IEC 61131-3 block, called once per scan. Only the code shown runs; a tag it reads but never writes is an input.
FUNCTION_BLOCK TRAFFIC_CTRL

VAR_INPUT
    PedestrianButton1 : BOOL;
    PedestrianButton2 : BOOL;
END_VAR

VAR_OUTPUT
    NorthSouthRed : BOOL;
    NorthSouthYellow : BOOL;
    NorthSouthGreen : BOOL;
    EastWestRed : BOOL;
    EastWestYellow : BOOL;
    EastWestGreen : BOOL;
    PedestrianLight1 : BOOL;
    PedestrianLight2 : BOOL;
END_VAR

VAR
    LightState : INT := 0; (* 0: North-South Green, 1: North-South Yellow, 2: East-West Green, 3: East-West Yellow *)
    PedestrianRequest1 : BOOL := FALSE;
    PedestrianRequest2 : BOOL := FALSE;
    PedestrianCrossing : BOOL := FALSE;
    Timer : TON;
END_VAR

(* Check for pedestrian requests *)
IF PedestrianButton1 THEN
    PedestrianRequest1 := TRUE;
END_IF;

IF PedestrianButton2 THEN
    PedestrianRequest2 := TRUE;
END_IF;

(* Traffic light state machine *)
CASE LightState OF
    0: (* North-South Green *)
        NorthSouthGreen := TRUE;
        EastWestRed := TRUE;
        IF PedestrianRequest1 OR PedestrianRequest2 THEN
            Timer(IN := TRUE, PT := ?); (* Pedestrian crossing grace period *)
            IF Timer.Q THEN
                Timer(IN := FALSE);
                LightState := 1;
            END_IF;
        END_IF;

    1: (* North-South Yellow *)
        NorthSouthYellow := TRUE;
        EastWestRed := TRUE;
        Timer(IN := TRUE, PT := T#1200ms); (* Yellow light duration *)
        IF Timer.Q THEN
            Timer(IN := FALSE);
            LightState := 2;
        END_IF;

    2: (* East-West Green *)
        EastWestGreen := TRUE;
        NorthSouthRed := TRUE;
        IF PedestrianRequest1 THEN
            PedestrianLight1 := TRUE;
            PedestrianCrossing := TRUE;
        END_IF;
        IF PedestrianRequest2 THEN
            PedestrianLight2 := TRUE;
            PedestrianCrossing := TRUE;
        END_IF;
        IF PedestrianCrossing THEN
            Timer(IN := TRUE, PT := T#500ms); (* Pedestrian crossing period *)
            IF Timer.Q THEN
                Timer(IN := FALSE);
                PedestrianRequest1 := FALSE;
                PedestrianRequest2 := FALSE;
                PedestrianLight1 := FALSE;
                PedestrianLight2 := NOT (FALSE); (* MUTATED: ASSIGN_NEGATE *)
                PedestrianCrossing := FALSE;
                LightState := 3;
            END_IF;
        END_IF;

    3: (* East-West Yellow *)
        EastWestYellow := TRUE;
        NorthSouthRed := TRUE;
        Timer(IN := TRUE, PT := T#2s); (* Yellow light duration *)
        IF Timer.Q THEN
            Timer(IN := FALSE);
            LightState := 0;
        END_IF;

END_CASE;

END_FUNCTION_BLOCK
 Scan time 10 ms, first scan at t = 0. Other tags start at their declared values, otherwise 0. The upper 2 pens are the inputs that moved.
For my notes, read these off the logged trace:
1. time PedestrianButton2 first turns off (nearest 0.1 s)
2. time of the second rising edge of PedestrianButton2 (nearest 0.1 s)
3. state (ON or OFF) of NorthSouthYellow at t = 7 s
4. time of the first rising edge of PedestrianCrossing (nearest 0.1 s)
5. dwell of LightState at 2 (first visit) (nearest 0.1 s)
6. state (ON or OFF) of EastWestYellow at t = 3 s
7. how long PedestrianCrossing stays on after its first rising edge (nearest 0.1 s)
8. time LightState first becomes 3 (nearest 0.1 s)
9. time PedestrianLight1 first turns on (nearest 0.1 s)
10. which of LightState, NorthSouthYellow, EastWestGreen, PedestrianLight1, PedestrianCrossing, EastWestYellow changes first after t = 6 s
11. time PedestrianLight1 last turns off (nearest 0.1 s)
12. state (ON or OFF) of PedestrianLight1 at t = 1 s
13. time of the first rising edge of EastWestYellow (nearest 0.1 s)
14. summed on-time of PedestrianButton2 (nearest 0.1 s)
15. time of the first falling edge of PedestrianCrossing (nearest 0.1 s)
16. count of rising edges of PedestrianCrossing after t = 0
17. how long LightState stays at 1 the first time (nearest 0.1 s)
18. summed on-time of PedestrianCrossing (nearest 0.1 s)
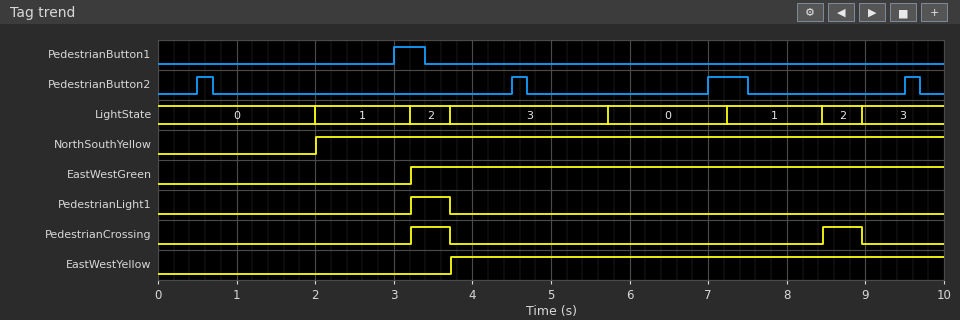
0.7 s
4.5 s
ON
3.2 s
0.5 s
OFF
0.5 s
3.7 s
3.2 s
LightState
3.7 s
OFF
3.7 s
1.1 s
3.7 s
2
1.2 s
1.0 s
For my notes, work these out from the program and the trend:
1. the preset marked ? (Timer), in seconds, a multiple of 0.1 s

1.5 s
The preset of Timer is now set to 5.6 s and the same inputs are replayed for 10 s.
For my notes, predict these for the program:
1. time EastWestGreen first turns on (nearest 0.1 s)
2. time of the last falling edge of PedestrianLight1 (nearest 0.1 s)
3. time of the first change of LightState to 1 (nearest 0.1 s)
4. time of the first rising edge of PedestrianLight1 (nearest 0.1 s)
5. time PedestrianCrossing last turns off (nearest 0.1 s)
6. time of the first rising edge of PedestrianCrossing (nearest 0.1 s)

7.3 s
7.8 s
6.1 s
7.3 s
7.8 s
7.3 s
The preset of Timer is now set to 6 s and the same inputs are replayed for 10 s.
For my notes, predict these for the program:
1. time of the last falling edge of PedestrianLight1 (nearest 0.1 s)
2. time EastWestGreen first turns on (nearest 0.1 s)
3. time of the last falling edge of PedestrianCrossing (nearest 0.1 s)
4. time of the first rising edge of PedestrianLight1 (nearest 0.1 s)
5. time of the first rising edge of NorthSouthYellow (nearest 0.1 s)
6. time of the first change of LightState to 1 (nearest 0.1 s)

8.2 s
7.7 s
8.2 s
7.7 s
6.5 s
6.5 s
